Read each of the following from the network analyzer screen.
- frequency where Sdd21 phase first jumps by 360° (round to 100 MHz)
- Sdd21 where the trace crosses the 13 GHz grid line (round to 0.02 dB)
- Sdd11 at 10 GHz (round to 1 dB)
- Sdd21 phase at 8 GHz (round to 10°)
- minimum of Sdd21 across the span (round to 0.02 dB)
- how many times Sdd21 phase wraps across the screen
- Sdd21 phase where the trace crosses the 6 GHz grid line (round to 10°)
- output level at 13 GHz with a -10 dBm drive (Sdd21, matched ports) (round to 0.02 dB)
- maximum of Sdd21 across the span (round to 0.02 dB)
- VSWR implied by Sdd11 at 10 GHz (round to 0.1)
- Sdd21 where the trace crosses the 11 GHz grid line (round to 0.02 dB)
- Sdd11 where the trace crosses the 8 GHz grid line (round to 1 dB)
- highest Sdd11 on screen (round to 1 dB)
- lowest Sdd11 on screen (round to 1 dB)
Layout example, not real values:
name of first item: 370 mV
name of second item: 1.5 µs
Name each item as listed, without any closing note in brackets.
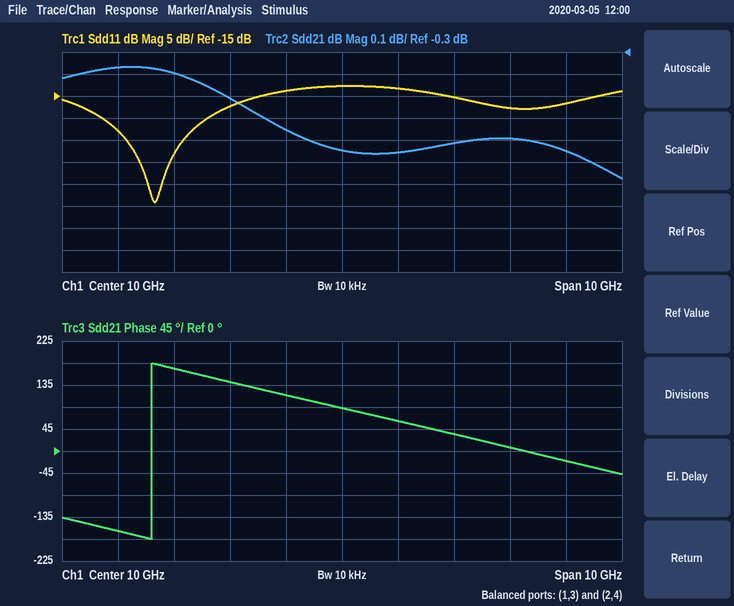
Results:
frequency where Sdd21 phase first jumps by 360°: 6.6 GHz
Sdd21 where the trace crosses the 13 GHz grid line: -0.70 dB
Sdd11 at 10 GHz: -13 dB
Sdd21 phase at 8 GHz: 140°
minimum of Sdd21 across the span: -0.88 dB
how many times Sdd21 phase wraps across the screen: 1
Sdd21 phase where the trace crosses the 6 GHz grid line: -160°
output level at 13 GHz with a -10 dBm drive (Sdd21, matched ports): -10.70 dBm
maximum of Sdd21 across the span: -0.36 dB
VSWR implied by Sdd11 at 10 GHz: 1.6
Sdd21 where the trace crosses the 11 GHz grid line: -0.76 dB
Sdd11 where the trace crosses the 8 GHz grid line: -17 dB
highest Sdd11 on screen: -13 dB
lowest Sdd11 on screen: -39 dB
